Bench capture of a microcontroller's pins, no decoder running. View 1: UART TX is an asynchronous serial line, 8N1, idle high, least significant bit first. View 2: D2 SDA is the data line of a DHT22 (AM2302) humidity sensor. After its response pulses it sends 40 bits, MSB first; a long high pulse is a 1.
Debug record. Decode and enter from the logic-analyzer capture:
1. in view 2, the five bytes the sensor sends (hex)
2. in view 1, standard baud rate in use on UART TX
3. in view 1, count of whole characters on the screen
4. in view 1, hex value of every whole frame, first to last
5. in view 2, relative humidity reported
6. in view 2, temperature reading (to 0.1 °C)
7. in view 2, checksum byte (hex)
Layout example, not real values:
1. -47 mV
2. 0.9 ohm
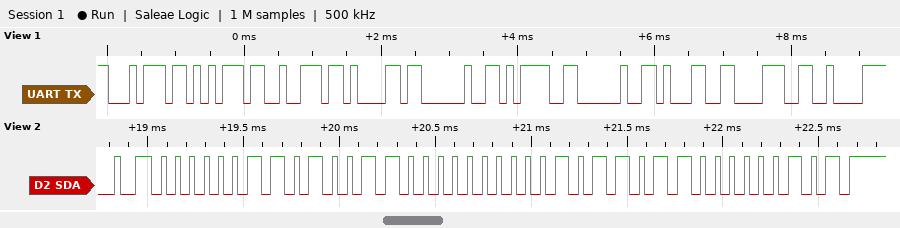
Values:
1. 03 4C 00 B6 05
2. 9600 baud
3. 10
4. 74 75 72 61 20 3D 20 31 38 C2
5. 84.4 %
6. 18.2 °C
7. 0x05
